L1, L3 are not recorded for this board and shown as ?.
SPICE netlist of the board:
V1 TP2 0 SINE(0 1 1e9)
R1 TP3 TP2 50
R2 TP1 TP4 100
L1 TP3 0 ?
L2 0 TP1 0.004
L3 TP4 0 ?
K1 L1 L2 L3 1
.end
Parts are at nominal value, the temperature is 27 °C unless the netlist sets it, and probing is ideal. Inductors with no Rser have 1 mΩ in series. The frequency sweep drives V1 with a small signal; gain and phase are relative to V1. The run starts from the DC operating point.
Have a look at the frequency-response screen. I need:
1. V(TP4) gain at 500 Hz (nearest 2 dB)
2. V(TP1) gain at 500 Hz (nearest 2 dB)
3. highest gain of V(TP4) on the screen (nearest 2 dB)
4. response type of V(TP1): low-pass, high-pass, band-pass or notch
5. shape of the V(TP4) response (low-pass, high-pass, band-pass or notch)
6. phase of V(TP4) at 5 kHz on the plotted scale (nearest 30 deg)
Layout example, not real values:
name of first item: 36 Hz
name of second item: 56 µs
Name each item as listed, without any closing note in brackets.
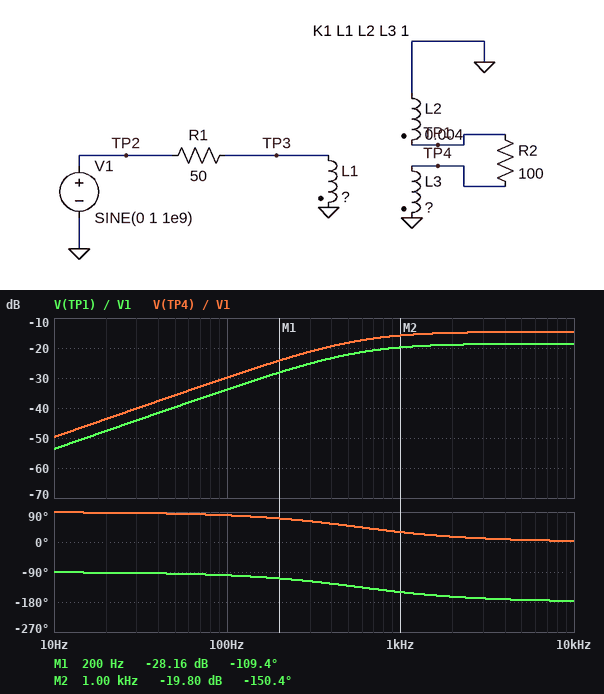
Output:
V(TP4) gain at 500 Hz: -18 dB
V(TP1) gain at 500 Hz: -22 dB
highest gain of V(TP4) on the screen: -14 dB
response type of V(TP1): low-pass, high-pass, band-pass or notch: high-pass
shape of the V(TP4) response: high-pass
phase of V(TP4) at 5 kHz on the plotted scale: 0 deg
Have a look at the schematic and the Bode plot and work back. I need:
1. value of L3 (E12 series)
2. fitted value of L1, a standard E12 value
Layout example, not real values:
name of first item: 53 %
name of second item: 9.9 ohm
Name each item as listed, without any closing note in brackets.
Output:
value of L3: 10 mH
fitted value of L1, a standard E12 value: 680 µH
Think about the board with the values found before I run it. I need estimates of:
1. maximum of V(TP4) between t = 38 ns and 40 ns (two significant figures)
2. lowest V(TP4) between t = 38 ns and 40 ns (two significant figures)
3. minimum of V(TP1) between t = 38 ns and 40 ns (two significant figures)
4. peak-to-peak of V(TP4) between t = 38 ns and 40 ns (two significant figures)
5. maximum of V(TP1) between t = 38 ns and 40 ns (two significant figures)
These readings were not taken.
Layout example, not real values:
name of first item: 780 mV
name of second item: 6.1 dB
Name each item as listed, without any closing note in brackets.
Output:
maximum of V(TP4) between t = 38 ns and 40 ns: 190 mV
lowest V(TP4) between t = 38 ns and 40 ns: -190 mV
minimum of V(TP1) between t = 38 ns and 40 ns: -120 mV
peak-to-peak of V(TP4) between t = 38 ns and 40 ns: 370 mV
maximum of V(TP1) between t = 38 ns and 40 ns: 120 mV
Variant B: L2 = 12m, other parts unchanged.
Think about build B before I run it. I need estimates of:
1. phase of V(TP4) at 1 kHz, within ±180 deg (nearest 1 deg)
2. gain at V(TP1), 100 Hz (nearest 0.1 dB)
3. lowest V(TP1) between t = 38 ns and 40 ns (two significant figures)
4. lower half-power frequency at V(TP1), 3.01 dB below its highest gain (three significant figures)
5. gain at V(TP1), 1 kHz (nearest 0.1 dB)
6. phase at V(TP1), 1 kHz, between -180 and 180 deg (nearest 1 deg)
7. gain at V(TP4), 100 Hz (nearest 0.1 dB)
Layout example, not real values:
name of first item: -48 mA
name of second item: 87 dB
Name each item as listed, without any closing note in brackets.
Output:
phase of V(TP4) at 1 kHz, within ±180 deg: 19 deg
gain at V(TP1), 100 Hz: -29.2 dB
lowest V(TP1) between t = 38 ns and 40 ns: -130 mV
lower half-power frequency at V(TP1), 3.01 dB below its highest gain: 352 Hz
gain at V(TP1), 1 kHz: -18.5 dB
phase at V(TP1), 1 kHz, between -180 and 180 deg: -161 deg
gain at V(TP4), 100 Hz: -30.0 dB
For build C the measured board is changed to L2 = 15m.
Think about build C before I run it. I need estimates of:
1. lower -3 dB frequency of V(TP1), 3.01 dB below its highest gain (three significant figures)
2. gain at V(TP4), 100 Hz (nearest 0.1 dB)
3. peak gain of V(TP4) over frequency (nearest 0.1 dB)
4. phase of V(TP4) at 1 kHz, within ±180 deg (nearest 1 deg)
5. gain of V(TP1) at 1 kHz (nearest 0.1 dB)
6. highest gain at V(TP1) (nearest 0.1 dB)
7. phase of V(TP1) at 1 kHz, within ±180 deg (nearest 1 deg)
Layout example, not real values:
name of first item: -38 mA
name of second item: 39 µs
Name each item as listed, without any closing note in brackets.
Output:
lower -3 dB frequency of V(TP1), 3.01 dB below its highest gain: 313 Hz
gain at V(TP4), 100 Hz: -30.1 dB
peak gain of V(TP4) over frequency: -19.8 dB
phase of V(TP4) at 1 kHz, within ±180 deg: 17 deg
gain of V(TP1) at 1 kHz: -18.4 dB
highest gain at V(TP1): -18.0 dB
phase of V(TP1) at 1 kHz, within ±180 deg: -163 deg
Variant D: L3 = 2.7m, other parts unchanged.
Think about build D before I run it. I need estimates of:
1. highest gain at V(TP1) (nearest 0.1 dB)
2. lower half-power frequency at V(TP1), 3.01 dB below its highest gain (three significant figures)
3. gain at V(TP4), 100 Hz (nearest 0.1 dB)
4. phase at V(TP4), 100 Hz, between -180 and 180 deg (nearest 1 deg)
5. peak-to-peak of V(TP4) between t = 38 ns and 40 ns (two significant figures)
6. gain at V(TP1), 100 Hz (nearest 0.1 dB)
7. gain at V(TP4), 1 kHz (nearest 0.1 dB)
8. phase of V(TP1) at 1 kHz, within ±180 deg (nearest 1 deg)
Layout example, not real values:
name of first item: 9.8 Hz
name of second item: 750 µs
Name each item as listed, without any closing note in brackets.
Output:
highest gain at V(TP1): -12.9 dB
lower half-power frequency at V(TP1), 3.01 dB below its highest gain: 1.09 kHz
gain at V(TP4), 100 Hz: -35.4 dB
phase at V(TP4), 100 Hz, between -180 and 180 deg: 85 deg
peak-to-peak of V(TP4) between t = 38 ns and 40 ns: 370 mV
gain at V(TP1), 100 Hz: -33.7 dB
gain at V(TP4), 1 kHz: -18.0 dB
phase of V(TP1) at 1 kHz, within ±180 deg: -133 deg
